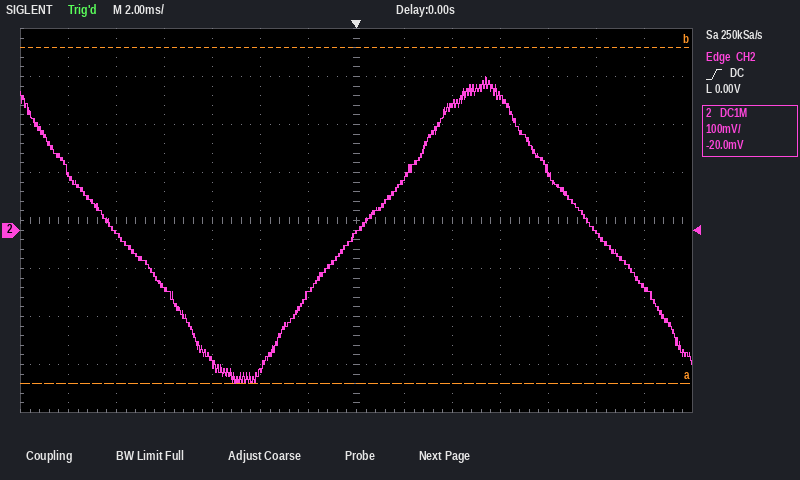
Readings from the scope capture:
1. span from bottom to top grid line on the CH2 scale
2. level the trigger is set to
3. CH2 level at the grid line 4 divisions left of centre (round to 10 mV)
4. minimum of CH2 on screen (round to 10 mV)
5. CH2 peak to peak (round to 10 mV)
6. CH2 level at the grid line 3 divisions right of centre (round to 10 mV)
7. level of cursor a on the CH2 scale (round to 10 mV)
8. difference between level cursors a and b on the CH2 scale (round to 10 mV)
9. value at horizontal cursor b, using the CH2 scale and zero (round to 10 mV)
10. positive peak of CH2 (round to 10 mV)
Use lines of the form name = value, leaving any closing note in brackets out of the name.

span from bottom to top grid line on the CH2 scale = 800 mV
level the trigger is set to = 0.00 V
CH2 level at the grid line 4 divisions left of centre = -120 mV
minimum of CH2 on screen = -320 mV
CH2 peak to peak = 640 mV
CH2 level at the grid line 3 divisions right of centre = 280 mV
level of cursor a on the CH2 scale = -320 mV
difference between level cursors a and b on the CH2 scale = 700 mV
value at horizontal cursor b, using the CH2 scale and zero = 380 mV
positive peak of CH2 = 320 mV
